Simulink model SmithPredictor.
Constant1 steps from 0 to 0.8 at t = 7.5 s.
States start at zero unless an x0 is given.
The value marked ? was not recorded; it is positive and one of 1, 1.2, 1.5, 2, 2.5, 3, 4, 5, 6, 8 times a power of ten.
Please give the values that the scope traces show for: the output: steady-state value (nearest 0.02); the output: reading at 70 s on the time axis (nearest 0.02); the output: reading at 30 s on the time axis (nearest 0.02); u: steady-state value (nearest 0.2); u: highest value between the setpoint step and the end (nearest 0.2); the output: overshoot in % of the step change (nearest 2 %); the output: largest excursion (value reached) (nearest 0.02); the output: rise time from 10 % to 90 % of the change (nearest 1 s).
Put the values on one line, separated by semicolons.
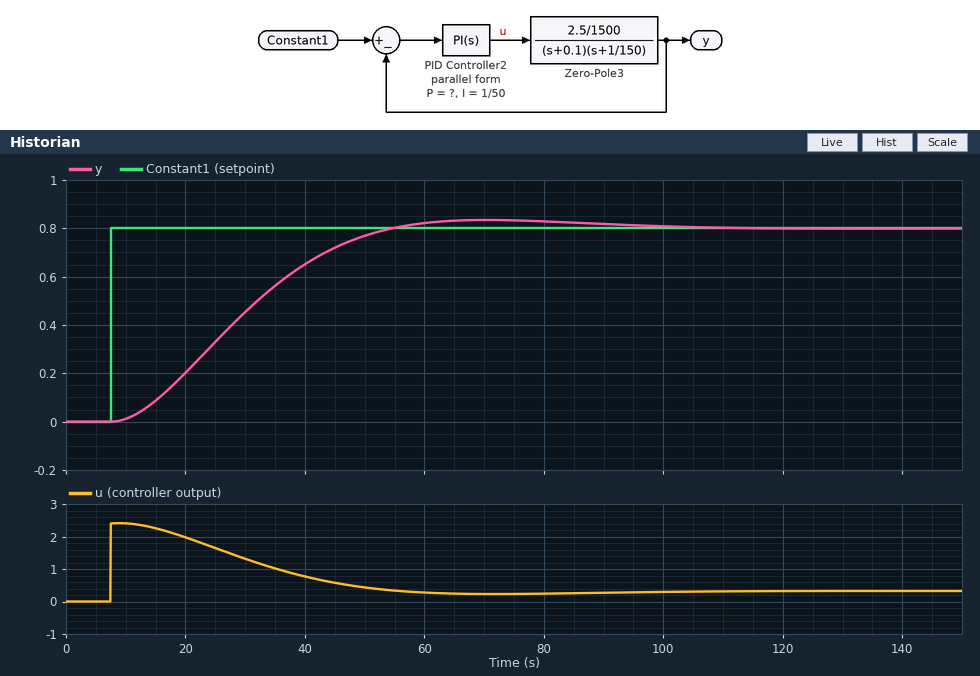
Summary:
0.80; 0.84; 0.46; 0.4; 2.4; 4 %; 0.84; 30 s
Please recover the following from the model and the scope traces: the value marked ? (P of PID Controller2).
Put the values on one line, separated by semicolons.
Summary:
3
